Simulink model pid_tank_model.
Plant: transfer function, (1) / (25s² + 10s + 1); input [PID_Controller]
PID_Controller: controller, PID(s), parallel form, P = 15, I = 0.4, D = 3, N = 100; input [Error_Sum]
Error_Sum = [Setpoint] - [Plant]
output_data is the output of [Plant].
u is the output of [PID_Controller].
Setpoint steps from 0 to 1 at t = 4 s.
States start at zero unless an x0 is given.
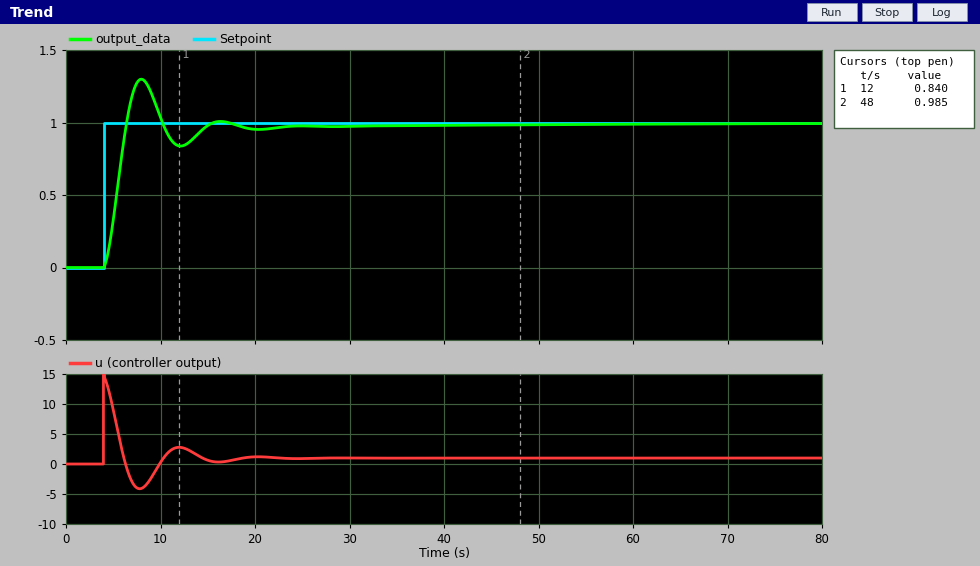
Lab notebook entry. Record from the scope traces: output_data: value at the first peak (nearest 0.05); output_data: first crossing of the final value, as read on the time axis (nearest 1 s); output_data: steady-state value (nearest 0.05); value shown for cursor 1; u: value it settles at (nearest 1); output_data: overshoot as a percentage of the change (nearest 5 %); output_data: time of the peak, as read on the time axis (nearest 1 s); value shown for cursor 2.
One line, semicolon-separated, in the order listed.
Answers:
1.30; 6 s; 1.00; 0.840; 1; 30 %; 8 s; 0.985
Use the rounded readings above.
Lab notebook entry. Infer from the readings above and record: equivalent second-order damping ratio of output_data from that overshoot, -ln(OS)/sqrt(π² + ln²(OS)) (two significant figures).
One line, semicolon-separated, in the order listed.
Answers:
0.36
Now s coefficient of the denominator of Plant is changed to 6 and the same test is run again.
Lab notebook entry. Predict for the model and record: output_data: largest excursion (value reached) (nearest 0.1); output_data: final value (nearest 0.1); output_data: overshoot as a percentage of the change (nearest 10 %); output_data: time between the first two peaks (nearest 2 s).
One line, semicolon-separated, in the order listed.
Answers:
1.4; 1.0; 40 %; 8 s
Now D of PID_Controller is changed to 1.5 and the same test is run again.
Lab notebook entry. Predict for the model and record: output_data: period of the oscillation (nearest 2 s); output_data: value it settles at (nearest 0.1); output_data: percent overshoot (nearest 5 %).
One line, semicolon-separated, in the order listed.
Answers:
8 s; 1.0; 35 %
